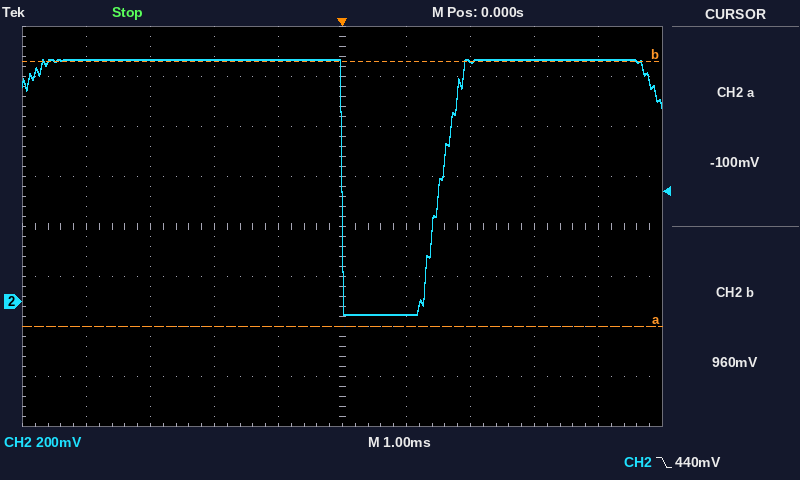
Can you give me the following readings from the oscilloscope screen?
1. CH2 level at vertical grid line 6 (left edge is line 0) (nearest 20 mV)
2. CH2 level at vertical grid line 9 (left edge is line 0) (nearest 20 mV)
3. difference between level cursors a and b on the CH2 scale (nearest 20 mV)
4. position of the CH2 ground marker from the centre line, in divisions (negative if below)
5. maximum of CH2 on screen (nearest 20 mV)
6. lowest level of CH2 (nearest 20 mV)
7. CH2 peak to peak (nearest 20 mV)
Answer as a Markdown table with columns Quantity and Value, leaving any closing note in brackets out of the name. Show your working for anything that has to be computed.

| Quantity | Value |
|---|---|
| CH2 level at vertical grid line 6 (left edge is line 0) | -60 mV |
| CH2 level at vertical grid line 9 (left edge is line 0) | 960 mV |
| difference between level cursors a and b on the CH2 scale | 1.06 V |
| position of the CH2 ground marker from the centre line, in divisions | -1.5 div |
| maximum of CH2 on screen | 960 mV |
| lowest level of CH2 | -60 mV |
| CH2 peak to peak | 960 mV − (-60 mV) = 1.02 V |
